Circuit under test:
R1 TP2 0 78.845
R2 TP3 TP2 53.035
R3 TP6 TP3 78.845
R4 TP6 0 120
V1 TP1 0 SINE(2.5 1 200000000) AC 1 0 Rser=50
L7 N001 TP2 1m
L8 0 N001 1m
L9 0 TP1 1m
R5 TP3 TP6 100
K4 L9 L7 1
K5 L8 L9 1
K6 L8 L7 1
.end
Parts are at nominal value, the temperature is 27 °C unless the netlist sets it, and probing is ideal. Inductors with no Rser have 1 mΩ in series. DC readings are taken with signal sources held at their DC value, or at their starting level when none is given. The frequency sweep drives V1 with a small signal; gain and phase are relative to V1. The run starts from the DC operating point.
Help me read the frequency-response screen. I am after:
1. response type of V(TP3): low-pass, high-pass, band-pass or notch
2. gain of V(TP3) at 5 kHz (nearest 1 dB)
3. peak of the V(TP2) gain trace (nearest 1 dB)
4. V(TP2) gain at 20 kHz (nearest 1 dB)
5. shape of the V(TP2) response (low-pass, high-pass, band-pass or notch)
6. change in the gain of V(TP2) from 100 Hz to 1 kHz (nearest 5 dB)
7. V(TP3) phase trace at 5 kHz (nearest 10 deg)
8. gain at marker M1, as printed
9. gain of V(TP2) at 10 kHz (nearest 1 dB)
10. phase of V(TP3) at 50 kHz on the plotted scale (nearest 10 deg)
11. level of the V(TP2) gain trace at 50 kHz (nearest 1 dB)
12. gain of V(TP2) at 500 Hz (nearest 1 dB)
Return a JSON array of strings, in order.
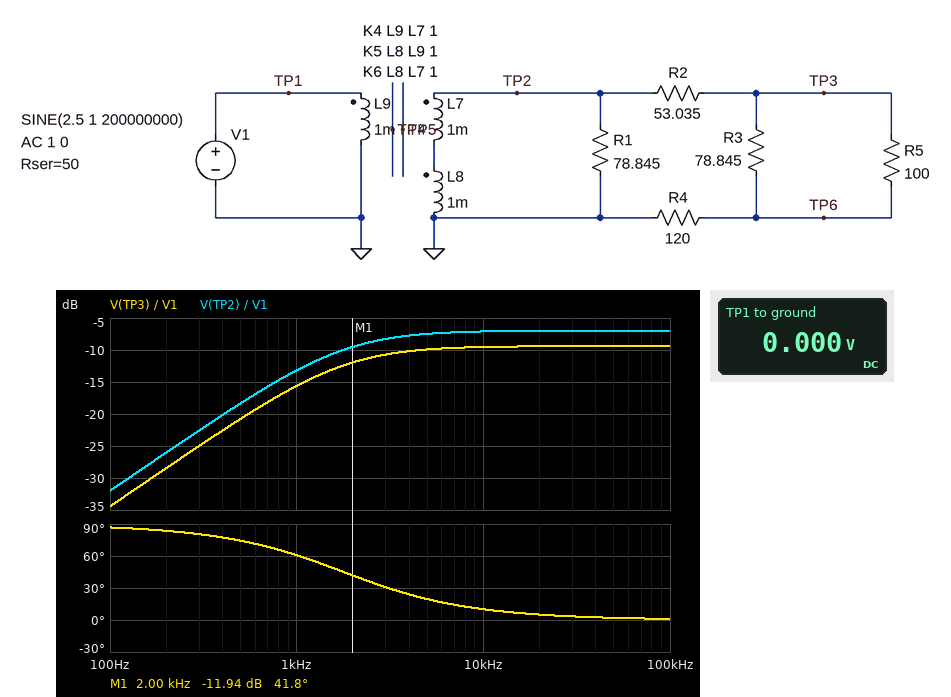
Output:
["high-pass", "-10 dB", "-7 dB", "-7 dB", "high-pass", "20 dB", "20 deg", "-11.94 dB", "-7 dB", "0 deg", "-7 dB", "-18 dB"]
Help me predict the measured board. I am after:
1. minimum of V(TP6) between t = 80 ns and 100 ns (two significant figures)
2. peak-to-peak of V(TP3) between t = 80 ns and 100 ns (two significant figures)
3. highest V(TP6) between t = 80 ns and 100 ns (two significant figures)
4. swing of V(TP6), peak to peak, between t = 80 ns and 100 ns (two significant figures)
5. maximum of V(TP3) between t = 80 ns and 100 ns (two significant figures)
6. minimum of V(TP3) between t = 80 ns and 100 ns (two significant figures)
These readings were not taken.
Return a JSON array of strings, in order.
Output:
["-250 mV", "680 mV", "250 mV", "500 mV", "340 mV", "-340 mV"]
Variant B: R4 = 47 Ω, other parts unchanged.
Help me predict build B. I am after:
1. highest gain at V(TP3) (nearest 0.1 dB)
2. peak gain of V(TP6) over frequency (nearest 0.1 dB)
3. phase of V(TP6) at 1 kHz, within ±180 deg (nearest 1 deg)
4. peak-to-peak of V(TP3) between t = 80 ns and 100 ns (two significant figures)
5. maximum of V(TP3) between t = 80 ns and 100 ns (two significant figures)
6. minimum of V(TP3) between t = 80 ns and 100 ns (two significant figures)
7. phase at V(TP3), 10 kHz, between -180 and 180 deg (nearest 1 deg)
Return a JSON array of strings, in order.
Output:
["-11.8 dB", "-17.6 dB", "58 deg", "510 mV", "260 mV", "-260 mV", "9 deg"]
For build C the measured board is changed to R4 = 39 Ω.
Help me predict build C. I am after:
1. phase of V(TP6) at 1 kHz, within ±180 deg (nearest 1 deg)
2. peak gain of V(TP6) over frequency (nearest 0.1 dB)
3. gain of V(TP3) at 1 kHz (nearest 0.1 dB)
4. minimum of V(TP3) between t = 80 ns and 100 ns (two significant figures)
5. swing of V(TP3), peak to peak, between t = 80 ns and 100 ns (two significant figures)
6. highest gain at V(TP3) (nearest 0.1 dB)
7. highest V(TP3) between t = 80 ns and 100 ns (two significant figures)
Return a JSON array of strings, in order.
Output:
["58 deg", "-18.8 dB", "-17.7 dB", "-240 mV", "490 mV", "-12.3 dB", "240 mV"]
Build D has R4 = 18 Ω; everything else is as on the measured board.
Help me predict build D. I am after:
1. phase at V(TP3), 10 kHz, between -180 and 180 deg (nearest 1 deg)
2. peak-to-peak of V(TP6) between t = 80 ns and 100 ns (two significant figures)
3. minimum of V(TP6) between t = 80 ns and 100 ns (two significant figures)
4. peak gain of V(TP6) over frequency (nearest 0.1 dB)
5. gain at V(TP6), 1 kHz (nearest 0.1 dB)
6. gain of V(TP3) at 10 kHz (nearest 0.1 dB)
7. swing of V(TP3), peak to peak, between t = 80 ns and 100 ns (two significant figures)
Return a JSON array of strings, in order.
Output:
["9 deg", "120 mV", "-59 mV", "-24.5 dB", "-29.7 dB", "-13.9 dB", "410 mV"]
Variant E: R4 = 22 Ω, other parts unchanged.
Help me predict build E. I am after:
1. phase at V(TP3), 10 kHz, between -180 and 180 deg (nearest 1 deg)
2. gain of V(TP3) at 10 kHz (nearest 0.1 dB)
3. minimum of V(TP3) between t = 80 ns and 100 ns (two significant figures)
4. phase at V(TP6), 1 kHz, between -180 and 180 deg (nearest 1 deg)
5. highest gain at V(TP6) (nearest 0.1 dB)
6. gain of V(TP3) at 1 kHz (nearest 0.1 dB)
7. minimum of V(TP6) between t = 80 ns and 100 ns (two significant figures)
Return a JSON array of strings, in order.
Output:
["9 deg", "-13.5 dB", "-210 mV", "57 deg", "-23.0 dB", "-18.7 dB", "-71 mV"]
